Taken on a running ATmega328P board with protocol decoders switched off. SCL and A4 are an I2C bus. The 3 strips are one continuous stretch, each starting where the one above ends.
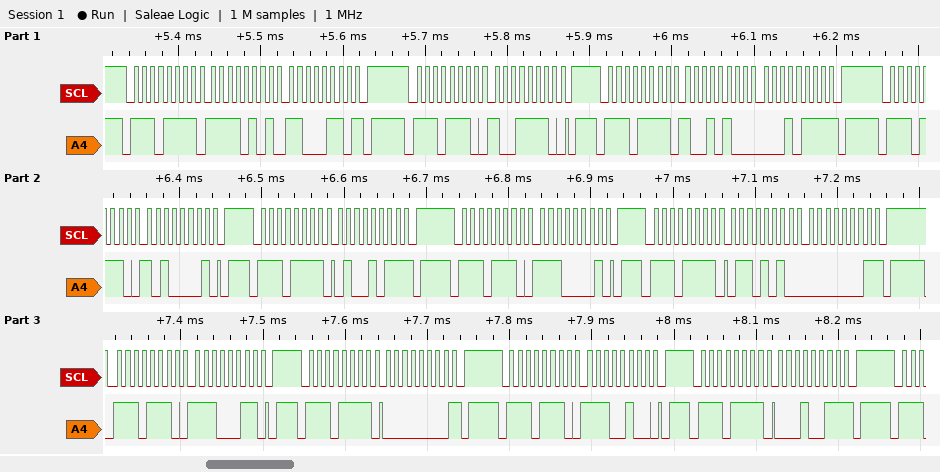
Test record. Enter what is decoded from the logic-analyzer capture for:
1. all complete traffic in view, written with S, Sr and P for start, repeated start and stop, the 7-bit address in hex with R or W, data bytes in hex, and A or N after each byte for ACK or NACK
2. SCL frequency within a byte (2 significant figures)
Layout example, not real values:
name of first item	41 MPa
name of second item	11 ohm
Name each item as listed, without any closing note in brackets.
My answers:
all complete traffic in view, written with S, Sr and P for start, repeated start and stop, the 7-bit address in hex with R or W, data bytes in hex, and A or N after each byte for ACK or NACK	S 77R A F5 A C6 N P S 77W A 9E A P S 77R A 94 A 17 N P S 77W A A1 A P S 77R A 4B N P S 77W A E1 A P S 77R A 6A A 01 N P S 77W A E3 A P S 77R A 00 N P S 77W A E4 A P S 77R A 13 N P
SCL frequency within a byte	100 kHz
